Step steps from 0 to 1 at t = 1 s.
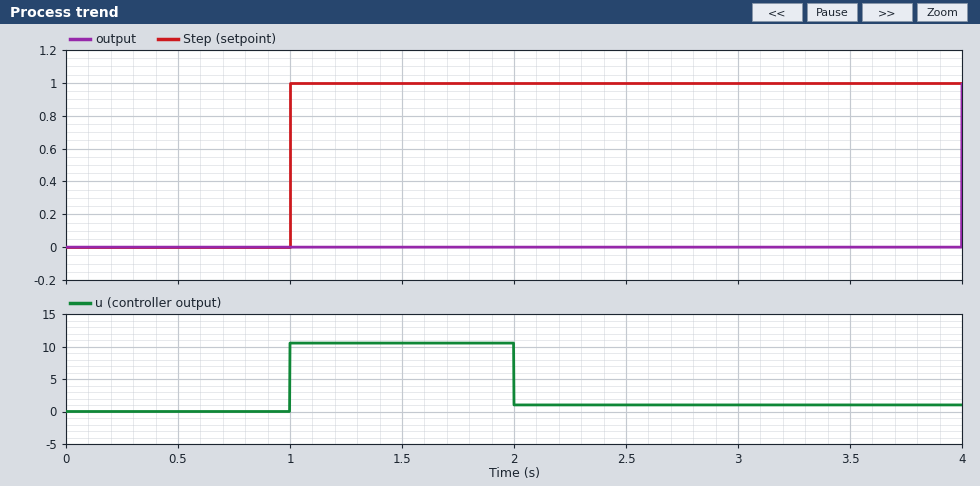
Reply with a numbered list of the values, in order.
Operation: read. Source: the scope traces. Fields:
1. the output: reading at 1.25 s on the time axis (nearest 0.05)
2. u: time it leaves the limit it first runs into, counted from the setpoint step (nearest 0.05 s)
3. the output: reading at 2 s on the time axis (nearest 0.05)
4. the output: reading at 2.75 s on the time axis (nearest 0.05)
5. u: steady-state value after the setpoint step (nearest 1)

1. 0.00
2. 1.00 s
3. 0.00
4. 0.00
5. 1
